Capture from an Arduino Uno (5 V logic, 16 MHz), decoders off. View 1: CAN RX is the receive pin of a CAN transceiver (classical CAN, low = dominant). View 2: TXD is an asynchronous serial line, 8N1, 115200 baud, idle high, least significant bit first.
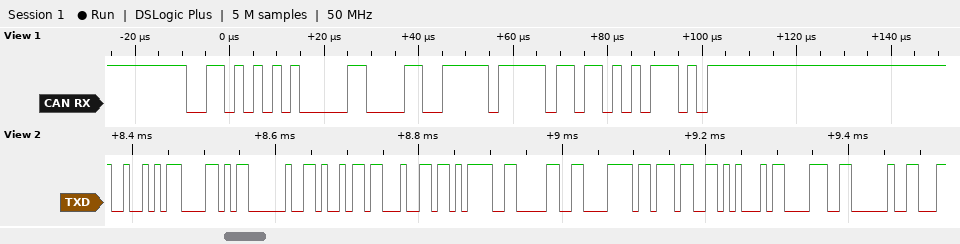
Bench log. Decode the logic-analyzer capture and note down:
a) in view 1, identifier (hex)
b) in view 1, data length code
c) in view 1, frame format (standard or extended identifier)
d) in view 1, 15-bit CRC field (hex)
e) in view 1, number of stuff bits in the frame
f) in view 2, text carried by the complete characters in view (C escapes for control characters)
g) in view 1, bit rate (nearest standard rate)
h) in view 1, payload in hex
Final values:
0x355
2
standard
0x76AE
3
"RX id=0x7E8 "
500 kbit/s
19 FF
